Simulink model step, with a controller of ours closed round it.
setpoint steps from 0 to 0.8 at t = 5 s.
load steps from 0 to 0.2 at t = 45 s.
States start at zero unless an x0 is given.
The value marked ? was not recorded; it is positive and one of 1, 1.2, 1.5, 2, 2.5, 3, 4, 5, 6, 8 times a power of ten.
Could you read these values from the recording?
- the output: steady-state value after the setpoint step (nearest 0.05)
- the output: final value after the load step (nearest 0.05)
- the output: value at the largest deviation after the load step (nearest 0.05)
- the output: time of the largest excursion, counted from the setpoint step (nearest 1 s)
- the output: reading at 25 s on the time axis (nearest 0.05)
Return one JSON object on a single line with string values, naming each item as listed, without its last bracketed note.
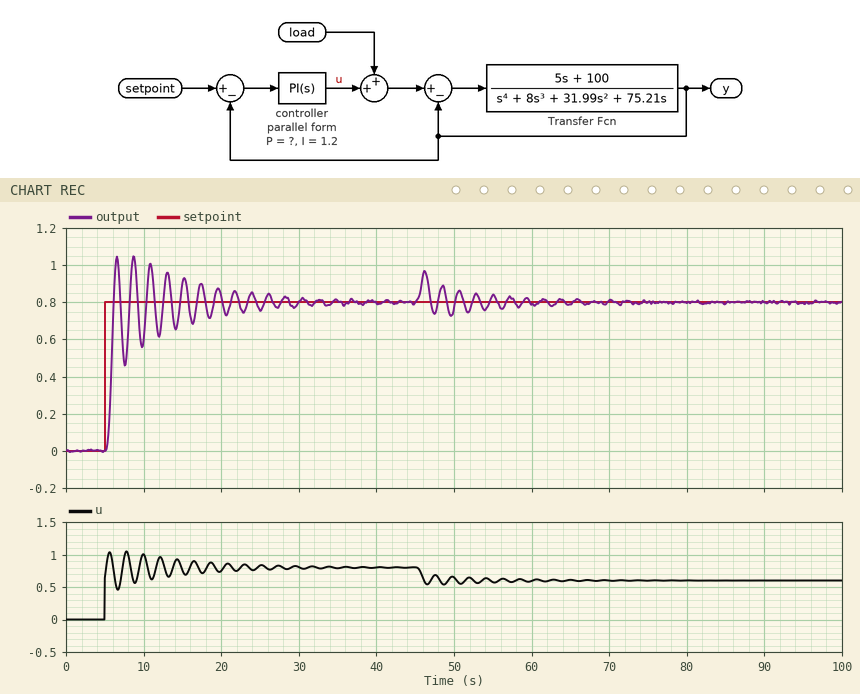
{"the output: steady-state value after the setpoint step": "0.80", "the output: final value after the load step": "0.80", "the output: value at the largest deviation after the load step": "0.95", "the output: time of the largest excursion, counted from the setpoint step": "4 s", "the output: reading at 25 s on the time axis": "0.75"}
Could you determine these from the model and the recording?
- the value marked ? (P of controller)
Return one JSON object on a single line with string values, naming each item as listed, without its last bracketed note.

{"the value marked ?": "0.8"}
